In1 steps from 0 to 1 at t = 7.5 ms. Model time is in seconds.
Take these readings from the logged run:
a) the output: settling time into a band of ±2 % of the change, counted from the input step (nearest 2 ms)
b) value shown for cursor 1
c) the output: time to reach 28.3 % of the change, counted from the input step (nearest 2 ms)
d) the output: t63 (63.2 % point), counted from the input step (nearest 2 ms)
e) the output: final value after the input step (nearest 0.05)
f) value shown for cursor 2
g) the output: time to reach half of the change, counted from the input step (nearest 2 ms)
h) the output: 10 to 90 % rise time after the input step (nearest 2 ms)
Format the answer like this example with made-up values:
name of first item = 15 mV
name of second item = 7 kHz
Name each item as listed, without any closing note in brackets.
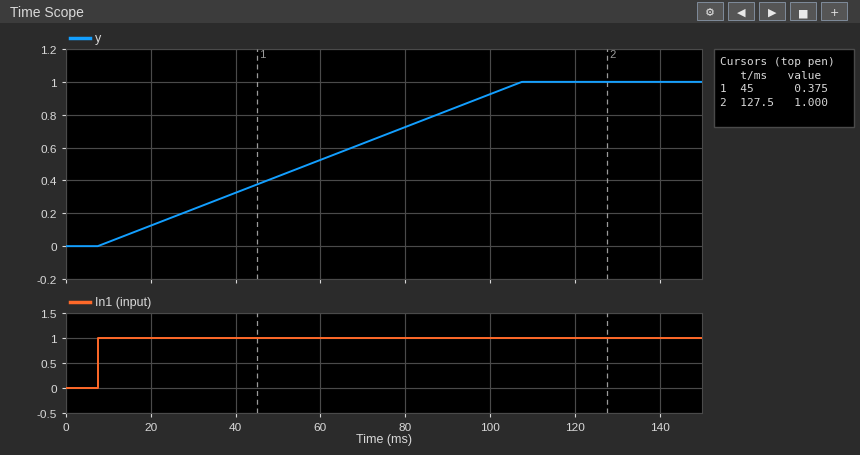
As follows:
the output: settling time into a band of ±2 % of the change, counted from the input step = 98 ms
value shown for cursor 1 = 0.375
the output: time to reach 28.3 % of the change, counted from the input step = 28 ms
the output: t63 (63.2 % point), counted from the input step = 64 ms
the output: final value after the input step = 1.00
value shown for cursor 2 = 1.000
the output: time to reach half of the change, counted from the input step = 50 ms
the output: 10 to 90 % rise time after the input step = 80 ms
